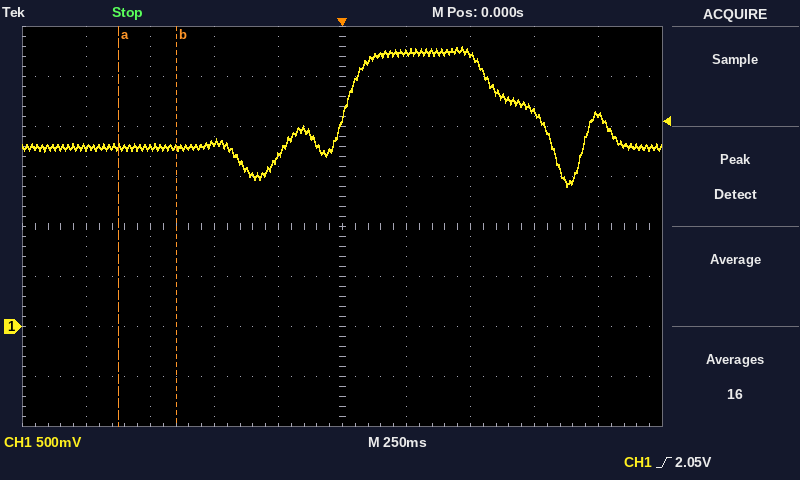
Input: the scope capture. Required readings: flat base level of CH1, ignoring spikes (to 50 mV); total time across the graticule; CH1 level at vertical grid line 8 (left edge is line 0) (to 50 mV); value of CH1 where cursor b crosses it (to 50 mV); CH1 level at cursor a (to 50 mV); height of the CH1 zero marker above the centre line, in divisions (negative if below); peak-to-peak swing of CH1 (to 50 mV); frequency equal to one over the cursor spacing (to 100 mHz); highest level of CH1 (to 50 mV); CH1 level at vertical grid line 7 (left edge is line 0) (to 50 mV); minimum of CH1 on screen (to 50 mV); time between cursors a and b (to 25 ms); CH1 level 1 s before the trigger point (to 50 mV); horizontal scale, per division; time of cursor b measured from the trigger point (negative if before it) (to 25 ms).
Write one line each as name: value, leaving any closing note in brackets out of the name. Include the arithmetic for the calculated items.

flat base level of CH1, ignoring spikes: 1.80 V
total time across the graticule: 2.5 s
CH1 level at vertical grid line 8 (left edge is line 0): 2.15 V
value of CH1 where cursor b crosses it: 1.80 V
CH1 level at cursor a: 1.80 V
height of the CH1 zero marker above the centre line, in divisions: -2.0 div
peak-to-peak swing of CH1: 2.80 V − (1.40 V) = 1.40 V
frequency equal to one over the cursor spacing: 1 / 225 ms ≈ 4.4 Hz
highest level of CH1: 2.80 V
CH1 level at vertical grid line 7 (left edge is line 0): 2.75 V
minimum of CH1 on screen: 1.40 V
time between cursors a and b: 225 ms
CH1 level 1 s before the trigger point: 1.80 V
horizontal scale, per division: 250 ms
time of cursor b measured from the trigger point (negative if before it): -650 ms
